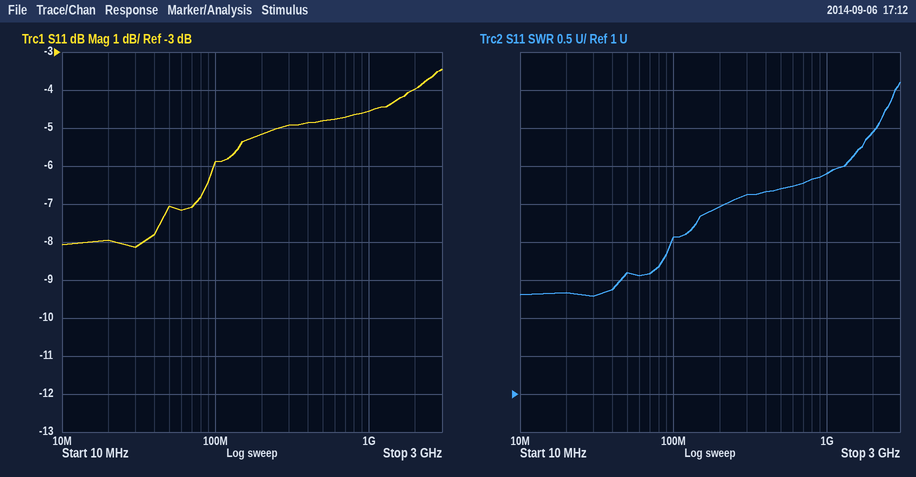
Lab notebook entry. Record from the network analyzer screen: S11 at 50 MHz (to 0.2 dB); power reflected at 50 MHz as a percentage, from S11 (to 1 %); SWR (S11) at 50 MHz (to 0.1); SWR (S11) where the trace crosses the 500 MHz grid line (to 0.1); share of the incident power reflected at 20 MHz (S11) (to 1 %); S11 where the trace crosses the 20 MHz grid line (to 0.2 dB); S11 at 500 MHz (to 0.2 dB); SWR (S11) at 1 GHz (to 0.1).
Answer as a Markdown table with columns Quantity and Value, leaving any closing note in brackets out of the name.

| Quantity | Value |
|---|---|
| S11 at 50 MHz | -7.0 dB |
| power reflected at 50 MHz as a percentage, from S11 | 20 % |
| SWR (S11) at 50 MHz | 2.6 |
| SWR (S11) where the trace crosses the 500 MHz grid line | 3.7 |
| share of the incident power reflected at 20 MHz (S11) | 16 % |
| S11 where the trace crosses the 20 MHz grid line | -8.0 dB |
| S11 at 500 MHz | -4.8 dB |
| SWR (S11) at 1 GHz | 3.9 |
